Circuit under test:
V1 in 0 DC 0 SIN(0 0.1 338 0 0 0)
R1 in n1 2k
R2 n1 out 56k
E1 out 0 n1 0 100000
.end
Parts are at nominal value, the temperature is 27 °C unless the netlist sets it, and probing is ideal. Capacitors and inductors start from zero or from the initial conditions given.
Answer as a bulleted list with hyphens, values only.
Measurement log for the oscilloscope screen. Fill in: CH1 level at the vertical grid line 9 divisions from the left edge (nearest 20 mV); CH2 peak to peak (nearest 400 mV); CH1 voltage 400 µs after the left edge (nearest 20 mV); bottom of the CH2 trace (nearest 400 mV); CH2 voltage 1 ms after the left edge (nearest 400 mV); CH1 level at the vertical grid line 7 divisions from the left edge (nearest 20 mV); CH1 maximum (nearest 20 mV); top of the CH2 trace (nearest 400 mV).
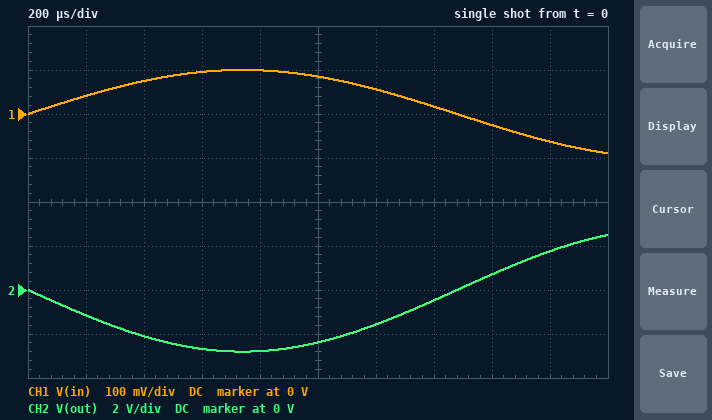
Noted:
- -60 mV
- 5.2 V
- 80 mV
- -2.8 V
- -2.4 V
- 20 mV
- 100 mV
- 2.4 V
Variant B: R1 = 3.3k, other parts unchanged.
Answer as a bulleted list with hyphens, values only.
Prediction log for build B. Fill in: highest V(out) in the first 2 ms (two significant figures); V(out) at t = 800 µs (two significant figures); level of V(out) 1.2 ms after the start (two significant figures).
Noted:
- 1.5 V
- -1.7 V
- -950 mV
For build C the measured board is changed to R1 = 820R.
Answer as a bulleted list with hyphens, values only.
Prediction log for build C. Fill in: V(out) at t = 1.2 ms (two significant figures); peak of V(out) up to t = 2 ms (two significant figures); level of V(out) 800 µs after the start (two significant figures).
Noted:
- -3.8 V
- 6.1 V
- -6.8 V
